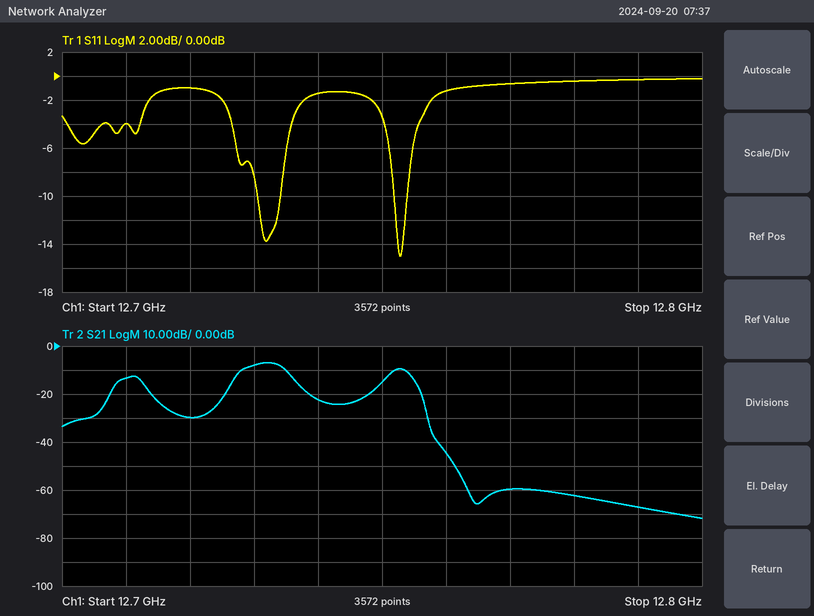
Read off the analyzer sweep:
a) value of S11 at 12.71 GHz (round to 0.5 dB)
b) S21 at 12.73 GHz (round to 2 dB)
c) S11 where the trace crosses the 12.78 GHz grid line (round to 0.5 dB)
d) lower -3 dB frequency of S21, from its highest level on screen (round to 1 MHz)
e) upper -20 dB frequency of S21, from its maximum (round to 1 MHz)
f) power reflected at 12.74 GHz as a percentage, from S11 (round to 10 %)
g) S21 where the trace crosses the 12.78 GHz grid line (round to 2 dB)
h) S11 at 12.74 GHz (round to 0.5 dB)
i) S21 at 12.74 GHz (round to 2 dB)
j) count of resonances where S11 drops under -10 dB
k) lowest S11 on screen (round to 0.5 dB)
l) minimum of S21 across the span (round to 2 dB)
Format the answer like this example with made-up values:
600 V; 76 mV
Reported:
-4.0 dB; -8 dB; -0.5 dB; 12.728 GHz; 12.757 GHz; 70 %; -62 dB; -1.5 dB; -22 dB; 2; -15.0 dB; -72 dB
